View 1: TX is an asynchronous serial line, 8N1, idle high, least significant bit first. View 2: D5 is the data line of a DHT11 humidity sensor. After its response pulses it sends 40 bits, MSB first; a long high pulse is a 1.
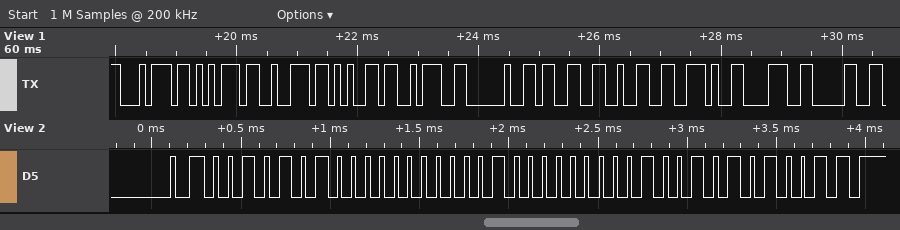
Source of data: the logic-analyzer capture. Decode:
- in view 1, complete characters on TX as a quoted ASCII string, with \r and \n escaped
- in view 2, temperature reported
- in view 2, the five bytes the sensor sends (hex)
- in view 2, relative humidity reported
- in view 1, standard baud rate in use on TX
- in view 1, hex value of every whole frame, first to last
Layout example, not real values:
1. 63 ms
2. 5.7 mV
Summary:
1. "ture: 32.80"
2. 32.9 °C
3. 2A 00 20 09 53
4. 42 %
5. 9600 baud
6. 74 75 72 65 3A 20 33 32 2E 38 30
